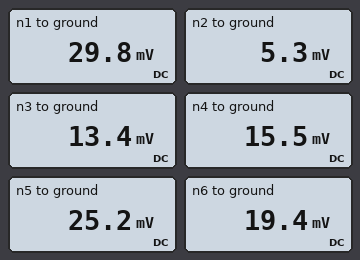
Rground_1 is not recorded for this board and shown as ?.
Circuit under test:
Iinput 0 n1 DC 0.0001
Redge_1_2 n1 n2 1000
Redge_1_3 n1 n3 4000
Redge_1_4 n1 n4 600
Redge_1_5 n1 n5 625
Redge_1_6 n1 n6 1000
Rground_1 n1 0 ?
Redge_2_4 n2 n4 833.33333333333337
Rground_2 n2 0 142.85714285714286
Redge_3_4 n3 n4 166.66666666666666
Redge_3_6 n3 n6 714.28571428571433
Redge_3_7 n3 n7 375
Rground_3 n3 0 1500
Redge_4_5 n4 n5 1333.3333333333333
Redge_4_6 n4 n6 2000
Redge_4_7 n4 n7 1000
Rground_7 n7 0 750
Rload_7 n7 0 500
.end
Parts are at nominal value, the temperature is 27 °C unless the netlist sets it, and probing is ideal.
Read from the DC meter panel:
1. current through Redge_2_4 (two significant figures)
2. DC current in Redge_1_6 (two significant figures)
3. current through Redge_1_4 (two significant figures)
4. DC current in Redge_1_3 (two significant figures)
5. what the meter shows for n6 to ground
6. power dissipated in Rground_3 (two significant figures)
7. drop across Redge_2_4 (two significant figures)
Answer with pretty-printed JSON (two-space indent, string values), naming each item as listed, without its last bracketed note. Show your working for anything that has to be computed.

{
  "current through Redge_2_4": "(15.5 mV - 5.3 mV) / 833.3 Ω = 12 µA",
  "DC current in Redge_1_6": "(29.8 mV - 19.4 mV) / 1 kΩ = 10 µA",
  "current through Redge_1_4": "(29.8 mV - 15.5 mV) / 600 Ω = 24 µA",
  "DC current in Redge_1_3": "(29.8 mV - 13.4 mV) / 4 kΩ = 4.1 µA",
  "what the meter shows for n6 to ground": "19.4 mV",
  "power dissipated in Rground_3": "(13.4 mV)^2 / 1.5 kΩ = 120 nW",
  "drop across Redge_2_4": "15.5 mV - 5.3 mV = 10 mV"
}
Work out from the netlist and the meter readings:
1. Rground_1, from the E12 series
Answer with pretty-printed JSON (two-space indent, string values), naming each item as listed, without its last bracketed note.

{
  "Rground_1, from the E12 series": "1 kΩ"
}
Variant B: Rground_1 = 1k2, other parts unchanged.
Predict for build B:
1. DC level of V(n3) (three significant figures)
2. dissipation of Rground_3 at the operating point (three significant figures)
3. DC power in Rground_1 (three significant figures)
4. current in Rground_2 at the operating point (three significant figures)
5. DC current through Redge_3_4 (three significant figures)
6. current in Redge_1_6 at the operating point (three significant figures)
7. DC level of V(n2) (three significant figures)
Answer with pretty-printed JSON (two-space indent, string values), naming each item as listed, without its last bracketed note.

{
  "DC level of V(n3)": "14.1 mV",
  "dissipation of Rground_3 at the operating point": "133 nW",
  "DC power in Rground_1": "820 nW",
  "current in Rground_2 at the operating point": "38.8 µA",
  "DC current through Redge_3_4": "13.3 µA",
  "current in Redge_1_6 at the operating point": "10.9 µA",
  "DC level of V(n2)": "5.54 mV"
}
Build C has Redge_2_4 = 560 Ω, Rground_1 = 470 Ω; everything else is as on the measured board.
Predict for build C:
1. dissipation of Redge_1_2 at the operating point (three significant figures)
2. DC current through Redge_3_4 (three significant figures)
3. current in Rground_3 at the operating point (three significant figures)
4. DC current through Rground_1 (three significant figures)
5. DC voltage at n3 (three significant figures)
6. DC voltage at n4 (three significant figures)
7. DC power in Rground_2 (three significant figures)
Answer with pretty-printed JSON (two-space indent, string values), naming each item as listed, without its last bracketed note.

{
  "dissipation of Redge_1_2 at the operating point": "316 nW",
  "DC current through Redge_3_4": "8.31 µA",
  "current in Rground_3 at the operating point": "6.32 µA",
  "DC current through Rground_1": "46.8 µA",
  "DC voltage at n3": "9.48 mV",
  "DC voltage at n4": "10.9 mV",
  "DC power in Rground_2": "125 nW"
}
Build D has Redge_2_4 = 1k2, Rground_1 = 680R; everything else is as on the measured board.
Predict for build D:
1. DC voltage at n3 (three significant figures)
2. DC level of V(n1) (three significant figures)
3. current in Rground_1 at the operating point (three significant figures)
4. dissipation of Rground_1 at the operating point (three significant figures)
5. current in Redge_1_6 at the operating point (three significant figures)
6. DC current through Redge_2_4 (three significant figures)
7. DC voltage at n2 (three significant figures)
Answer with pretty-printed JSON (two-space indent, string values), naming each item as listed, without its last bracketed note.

{
  "DC voltage at n3": "12.3 mV",
  "DC level of V(n1)": "26.5 mV",
  "current in Rground_1 at the operating point": "38.9 µA",
  "dissipation of Rground_1 at the operating point": "1.03 µW",
  "current in Redge_1_6 at the operating point": "8.94 µA",
  "DC current through Redge_2_4": "8.31 µA",
  "DC voltage at n2": "4.35 mV"
}
